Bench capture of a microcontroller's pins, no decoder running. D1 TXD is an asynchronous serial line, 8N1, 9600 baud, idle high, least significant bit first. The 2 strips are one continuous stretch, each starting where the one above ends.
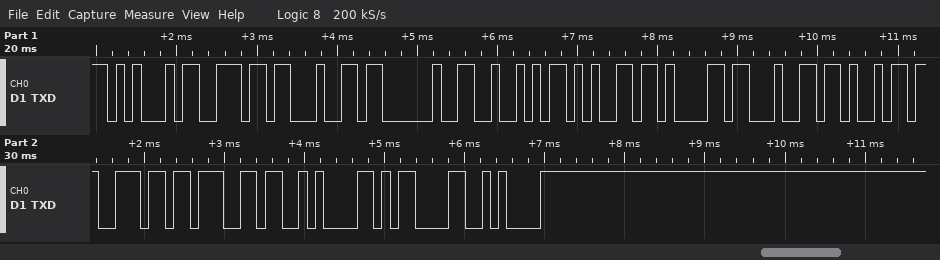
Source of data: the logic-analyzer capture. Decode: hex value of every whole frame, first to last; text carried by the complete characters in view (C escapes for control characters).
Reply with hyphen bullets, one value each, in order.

- 0x45 0x6E 0x64 0x20 0x52 0x65 0x61 0x64 0x69 0x6E 0x67 0x0A 0x0D 0x0A
- "End Reading\n\r\n"
